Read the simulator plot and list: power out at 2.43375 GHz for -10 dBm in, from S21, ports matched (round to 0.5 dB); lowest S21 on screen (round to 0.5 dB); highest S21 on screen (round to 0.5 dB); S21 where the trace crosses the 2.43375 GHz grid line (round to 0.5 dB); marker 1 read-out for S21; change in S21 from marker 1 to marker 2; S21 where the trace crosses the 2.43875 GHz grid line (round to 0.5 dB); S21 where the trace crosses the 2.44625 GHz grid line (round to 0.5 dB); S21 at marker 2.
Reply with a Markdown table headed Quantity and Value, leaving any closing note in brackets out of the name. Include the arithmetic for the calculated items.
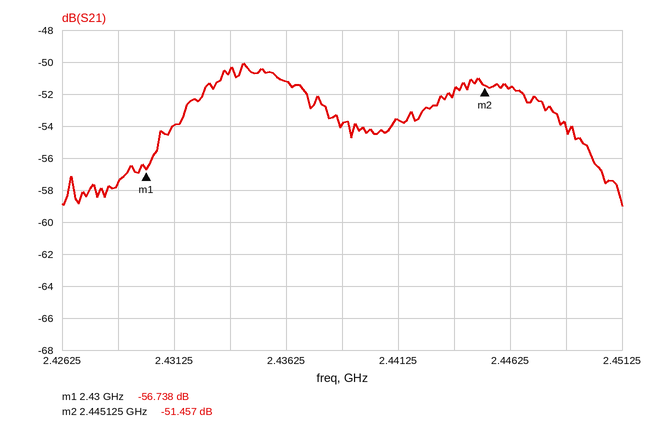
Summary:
| Quantity | Value |
|---|---|
| power out at 2.43375 GHz for -10 dBm in, from S21, ports matched | -10 dBm + (-50.5 dB) = -60.5 dBm |
| lowest S21 on screen | -59.0 dB |
| highest S21 on screen | -50.0 dB |
| S21 where the trace crosses the 2.43375 GHz grid line | -50.5 dB |
| marker 1 read-out for S21 | -56.738 dB |
| change in S21 from marker 1 to marker 2 | -51.457 − (-56.738) = 5.281 dB |
| S21 where the trace crosses the 2.43875 GHz grid line | -54.0 dB |
| S21 where the trace crosses the 2.44625 GHz grid line | -51.5 dB |
| S21 at marker 2 | -51.457 dB |
